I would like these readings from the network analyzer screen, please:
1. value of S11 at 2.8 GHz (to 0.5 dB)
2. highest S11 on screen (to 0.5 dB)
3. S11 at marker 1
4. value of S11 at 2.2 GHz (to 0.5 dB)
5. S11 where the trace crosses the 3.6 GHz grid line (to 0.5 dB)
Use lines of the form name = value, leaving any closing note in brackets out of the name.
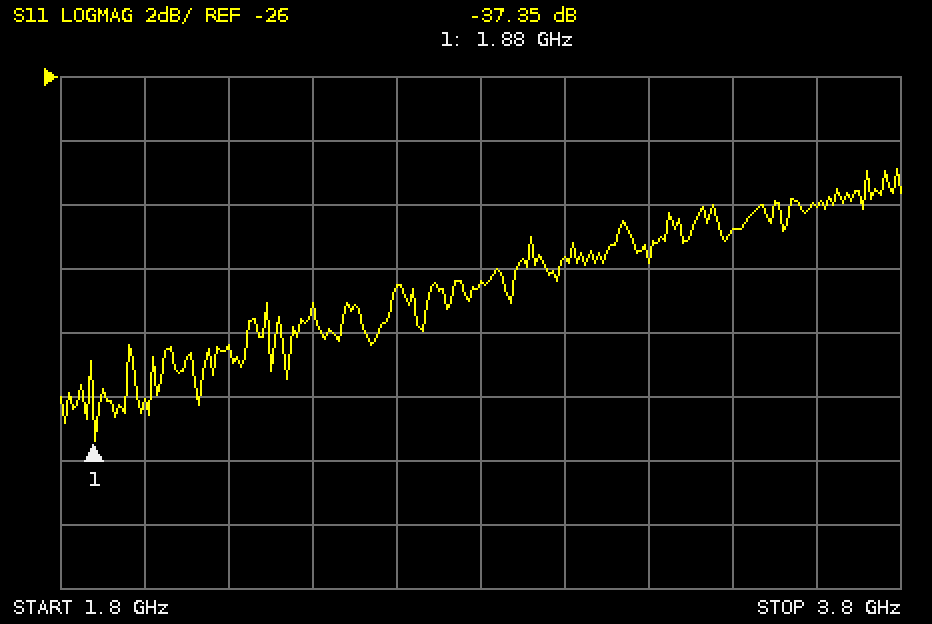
value of S11 at 2.8 GHz = -32.5 dB
highest S11 on screen = -29.0 dB
S11 at marker 1 = -37.35 dB
value of S11 at 2.2 GHz = -34.5 dB
S11 where the trace crosses the 3.6 GHz grid line = -30.0 dB
